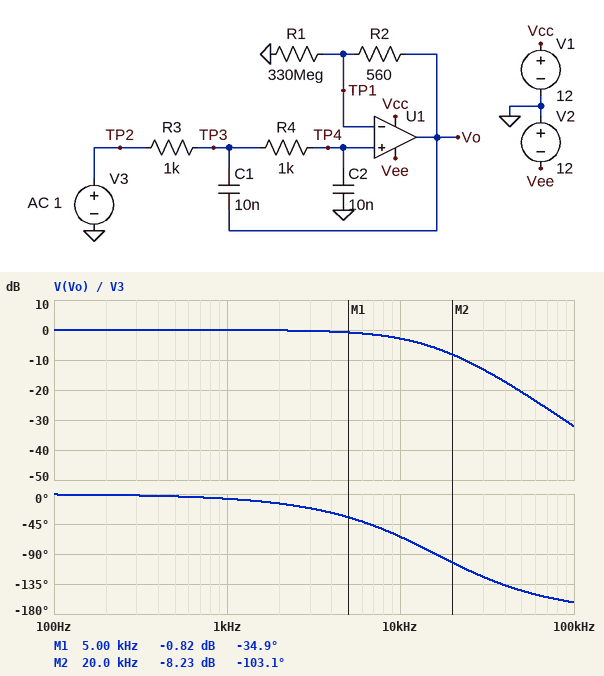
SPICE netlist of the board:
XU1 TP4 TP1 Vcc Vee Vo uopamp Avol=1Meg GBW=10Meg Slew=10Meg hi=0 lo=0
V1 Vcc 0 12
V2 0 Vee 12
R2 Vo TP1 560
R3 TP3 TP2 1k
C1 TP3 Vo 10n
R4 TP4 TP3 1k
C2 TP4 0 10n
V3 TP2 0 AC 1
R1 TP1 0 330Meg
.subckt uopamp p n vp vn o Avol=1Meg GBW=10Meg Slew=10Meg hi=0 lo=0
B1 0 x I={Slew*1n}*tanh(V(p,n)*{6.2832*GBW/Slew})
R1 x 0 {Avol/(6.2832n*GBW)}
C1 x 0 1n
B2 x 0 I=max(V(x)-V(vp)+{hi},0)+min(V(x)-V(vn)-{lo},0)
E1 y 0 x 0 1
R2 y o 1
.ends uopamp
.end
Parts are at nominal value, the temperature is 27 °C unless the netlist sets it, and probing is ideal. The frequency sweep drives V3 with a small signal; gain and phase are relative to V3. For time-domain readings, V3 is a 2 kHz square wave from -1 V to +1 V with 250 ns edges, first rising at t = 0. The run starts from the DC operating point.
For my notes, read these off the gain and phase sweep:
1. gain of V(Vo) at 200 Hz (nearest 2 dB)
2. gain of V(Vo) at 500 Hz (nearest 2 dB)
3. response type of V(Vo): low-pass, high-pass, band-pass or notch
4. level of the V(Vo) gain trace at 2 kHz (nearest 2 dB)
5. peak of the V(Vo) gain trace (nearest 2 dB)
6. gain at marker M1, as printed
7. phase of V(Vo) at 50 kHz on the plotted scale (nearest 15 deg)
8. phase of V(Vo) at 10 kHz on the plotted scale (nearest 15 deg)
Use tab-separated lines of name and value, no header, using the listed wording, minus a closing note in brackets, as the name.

gain of V(Vo) at 200 Hz	0 dB
gain of V(Vo) at 500 Hz	0 dB
response type of V(Vo): low-pass, high-pass, band-pass or notch	low-pass
level of the V(Vo) gain trace at 2 kHz	0 dB
peak of the V(Vo) gain trace	0 dB
gain at marker M1, as printed	-0.82 dB
phase of V(Vo) at 50 kHz on the plotted scale	-150 deg
phase of V(Vo) at 10 kHz on the plotted scale	-60 deg
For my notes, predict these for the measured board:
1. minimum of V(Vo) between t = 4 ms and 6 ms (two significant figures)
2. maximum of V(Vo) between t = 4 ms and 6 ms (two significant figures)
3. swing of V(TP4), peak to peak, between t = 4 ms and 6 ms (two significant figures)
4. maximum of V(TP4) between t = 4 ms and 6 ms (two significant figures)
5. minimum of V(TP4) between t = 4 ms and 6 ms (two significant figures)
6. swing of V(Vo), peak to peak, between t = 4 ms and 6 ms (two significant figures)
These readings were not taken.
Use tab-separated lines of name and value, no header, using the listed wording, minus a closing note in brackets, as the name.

minimum of V(Vo) between t = 4 ms and 6 ms	-1.0 V
maximum of V(Vo) between t = 4 ms and 6 ms	1.0 V
swing of V(TP4), peak to peak, between t = 4 ms and 6 ms	2.0 V
maximum of V(TP4) between t = 4 ms and 6 ms	1.0 V
minimum of V(TP4) between t = 4 ms and 6 ms	-1.0 V
swing of V(Vo), peak to peak, between t = 4 ms and 6 ms	2.0 V
